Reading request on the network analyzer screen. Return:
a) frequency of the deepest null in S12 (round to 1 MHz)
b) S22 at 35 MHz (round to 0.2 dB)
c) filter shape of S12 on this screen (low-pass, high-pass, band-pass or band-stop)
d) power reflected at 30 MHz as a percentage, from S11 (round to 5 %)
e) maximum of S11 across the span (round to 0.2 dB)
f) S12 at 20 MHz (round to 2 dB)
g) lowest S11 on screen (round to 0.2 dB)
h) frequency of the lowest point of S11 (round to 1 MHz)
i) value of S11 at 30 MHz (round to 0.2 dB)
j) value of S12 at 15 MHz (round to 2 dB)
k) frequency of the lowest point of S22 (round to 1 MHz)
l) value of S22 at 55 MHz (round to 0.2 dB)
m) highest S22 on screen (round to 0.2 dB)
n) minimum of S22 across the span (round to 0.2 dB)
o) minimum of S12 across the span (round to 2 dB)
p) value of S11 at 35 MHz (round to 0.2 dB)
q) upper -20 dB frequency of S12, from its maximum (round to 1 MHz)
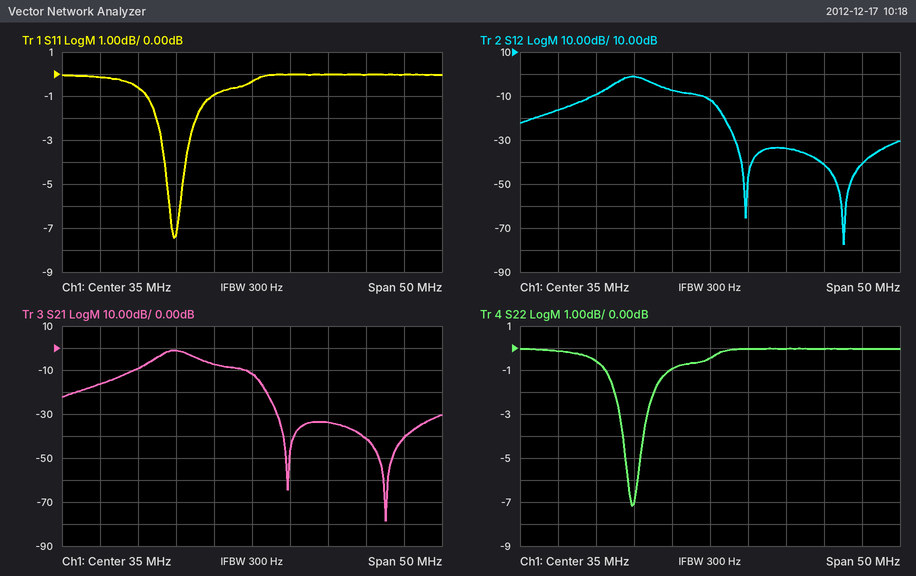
53 MHz
-0.4 dB
band-pass
80 %
0.0 dB
-10 dB
-7.4 dB
25 MHz
-1.0 dB
-16 dB
25 MHz
0.0 dB
0.0 dB
-7.2 dB
-78 dB
-0.4 dB
37 MHz
